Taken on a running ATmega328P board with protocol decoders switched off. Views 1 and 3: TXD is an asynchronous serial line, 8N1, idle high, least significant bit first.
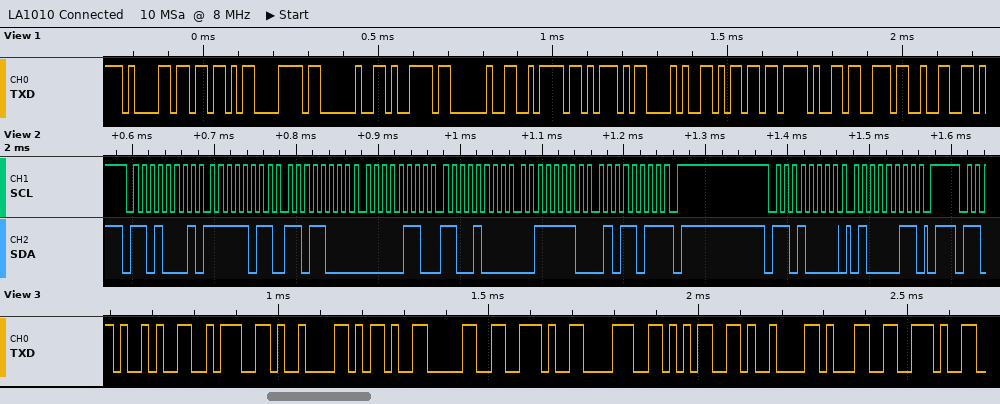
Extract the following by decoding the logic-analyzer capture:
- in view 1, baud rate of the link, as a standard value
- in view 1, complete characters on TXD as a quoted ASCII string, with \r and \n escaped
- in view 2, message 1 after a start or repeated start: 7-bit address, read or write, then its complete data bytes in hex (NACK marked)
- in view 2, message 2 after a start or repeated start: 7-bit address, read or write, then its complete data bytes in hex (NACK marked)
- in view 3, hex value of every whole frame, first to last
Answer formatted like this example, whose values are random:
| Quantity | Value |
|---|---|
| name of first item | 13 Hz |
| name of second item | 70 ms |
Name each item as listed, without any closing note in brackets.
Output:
| Quantity | Value |
|---|---|
| in view 1, baud rate of the link, as a standard value | 57600 baud |
| in view 1, complete characters on TXD as a quoted ASCII string, with \r and \n escaped | "a[x y z](m/s2" |
| in view 2, message 1 after a start or repeated start: 7-bit address, read or write, then its complete data bytes in hex | 0x68 read: FB D8 06 C8 3E 5B NACK |
| in view 2, message 2 after a start or repeated start: 7-bit address, read or write, then its complete data bytes in hex | 0x68 write: 43 |
| in view 3, hex value of every whole frame, first to last | 29 3A 09 2D 30 2E 38 35 09 31 2E |
